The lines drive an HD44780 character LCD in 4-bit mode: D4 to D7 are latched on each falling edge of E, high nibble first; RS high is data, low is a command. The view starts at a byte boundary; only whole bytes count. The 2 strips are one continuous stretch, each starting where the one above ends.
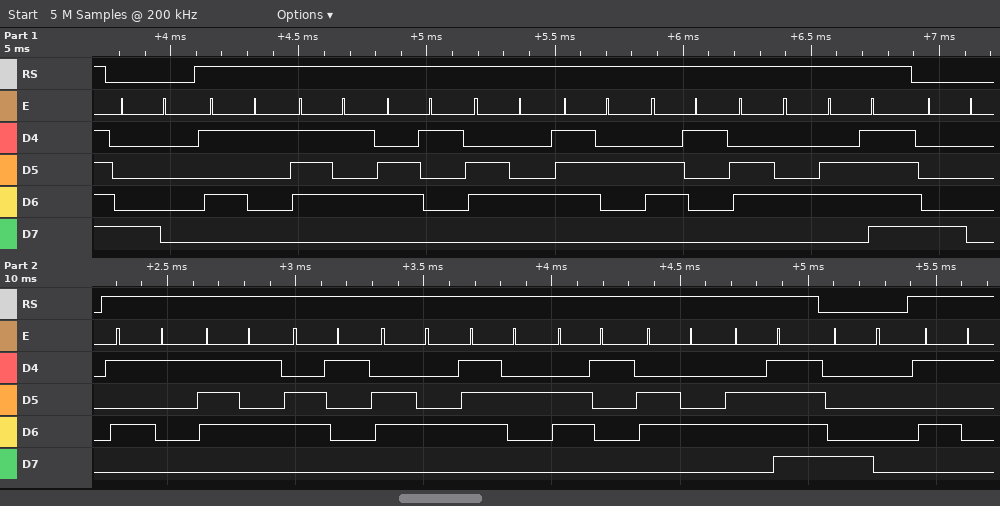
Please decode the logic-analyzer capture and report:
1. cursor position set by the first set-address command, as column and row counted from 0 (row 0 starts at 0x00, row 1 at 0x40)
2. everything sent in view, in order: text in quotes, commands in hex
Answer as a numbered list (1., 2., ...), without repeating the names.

1. column 0, row 0
2. 0x80 "Quadrado" 0x80 "Quadrado" 0x80 "Q"
